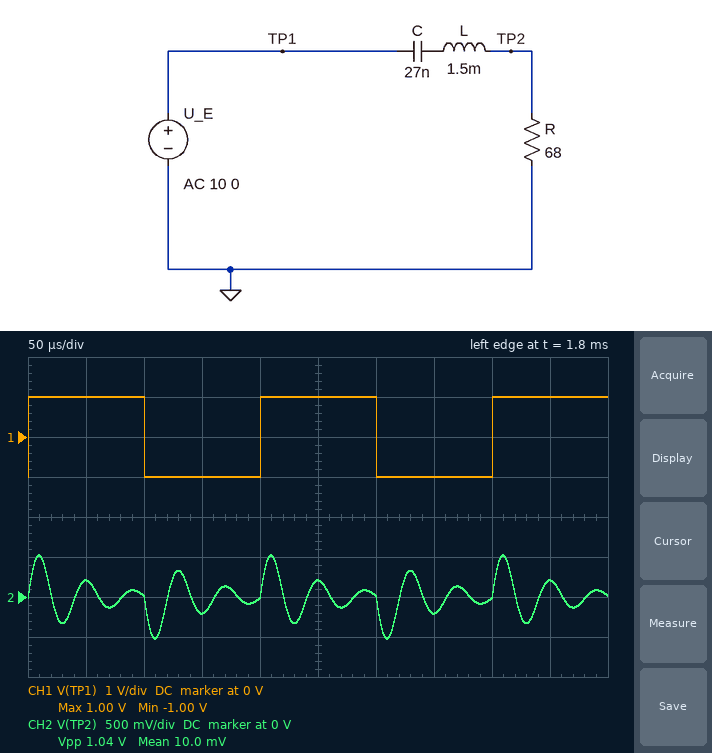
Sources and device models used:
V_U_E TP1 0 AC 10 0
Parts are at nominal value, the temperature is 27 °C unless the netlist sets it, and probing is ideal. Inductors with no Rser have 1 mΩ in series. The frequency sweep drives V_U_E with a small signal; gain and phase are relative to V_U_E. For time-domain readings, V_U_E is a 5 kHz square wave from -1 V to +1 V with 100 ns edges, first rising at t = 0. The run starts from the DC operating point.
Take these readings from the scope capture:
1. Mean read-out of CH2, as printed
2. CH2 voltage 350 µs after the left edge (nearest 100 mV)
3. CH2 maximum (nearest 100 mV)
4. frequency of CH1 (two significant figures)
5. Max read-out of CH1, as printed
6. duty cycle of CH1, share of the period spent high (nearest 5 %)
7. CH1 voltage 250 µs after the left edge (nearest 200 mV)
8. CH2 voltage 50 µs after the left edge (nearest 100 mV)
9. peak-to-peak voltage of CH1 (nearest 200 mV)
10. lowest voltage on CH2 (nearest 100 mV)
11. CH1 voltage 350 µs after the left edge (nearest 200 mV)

10.0 mV
-200 mV
500 mV
5.0 kHz
1.00 V
50 %
1.0 V
200 mV
2.0 V
-500 mV
-1.0 V
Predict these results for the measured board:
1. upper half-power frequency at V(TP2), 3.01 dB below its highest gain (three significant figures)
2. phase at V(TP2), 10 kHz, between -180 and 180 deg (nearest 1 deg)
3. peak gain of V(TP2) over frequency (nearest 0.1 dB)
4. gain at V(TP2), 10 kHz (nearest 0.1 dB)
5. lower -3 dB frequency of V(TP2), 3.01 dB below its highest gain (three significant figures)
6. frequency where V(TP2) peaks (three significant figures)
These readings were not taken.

28.9 kHz
82 deg
0 dB
-17.3 dB
21.7 kHz
25.0 kHz
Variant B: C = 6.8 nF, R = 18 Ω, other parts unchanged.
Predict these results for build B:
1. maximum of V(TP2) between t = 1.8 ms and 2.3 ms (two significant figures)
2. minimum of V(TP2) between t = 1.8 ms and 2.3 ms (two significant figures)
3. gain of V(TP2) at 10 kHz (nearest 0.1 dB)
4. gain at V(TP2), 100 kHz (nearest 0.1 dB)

48 mV
-48 mV
-41.9 dB
-31.9 dB
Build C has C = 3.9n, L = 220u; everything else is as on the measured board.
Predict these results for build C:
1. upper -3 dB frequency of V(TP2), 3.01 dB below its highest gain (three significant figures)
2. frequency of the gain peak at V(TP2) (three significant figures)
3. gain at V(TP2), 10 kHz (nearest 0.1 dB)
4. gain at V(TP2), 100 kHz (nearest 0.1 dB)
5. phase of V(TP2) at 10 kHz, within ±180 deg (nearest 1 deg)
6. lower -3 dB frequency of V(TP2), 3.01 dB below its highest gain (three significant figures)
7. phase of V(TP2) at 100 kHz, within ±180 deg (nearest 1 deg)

198 kHz
172 kHz
-35.5 dB
-12.2 dB
89 deg
149 kHz
76 deg
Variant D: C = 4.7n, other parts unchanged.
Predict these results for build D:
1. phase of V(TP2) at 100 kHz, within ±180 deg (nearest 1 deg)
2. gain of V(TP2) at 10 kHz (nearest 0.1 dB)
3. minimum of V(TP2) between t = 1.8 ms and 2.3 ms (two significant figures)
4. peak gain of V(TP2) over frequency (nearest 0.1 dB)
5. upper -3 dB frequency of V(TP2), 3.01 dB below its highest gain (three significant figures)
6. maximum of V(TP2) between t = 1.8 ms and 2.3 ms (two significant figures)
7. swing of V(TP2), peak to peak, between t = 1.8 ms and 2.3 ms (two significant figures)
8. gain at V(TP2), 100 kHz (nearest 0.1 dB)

-84 deg
-33.7 dB
-200 mV
0 dB
63.7 kHz
200 mV
400 mV
-19.0 dB
